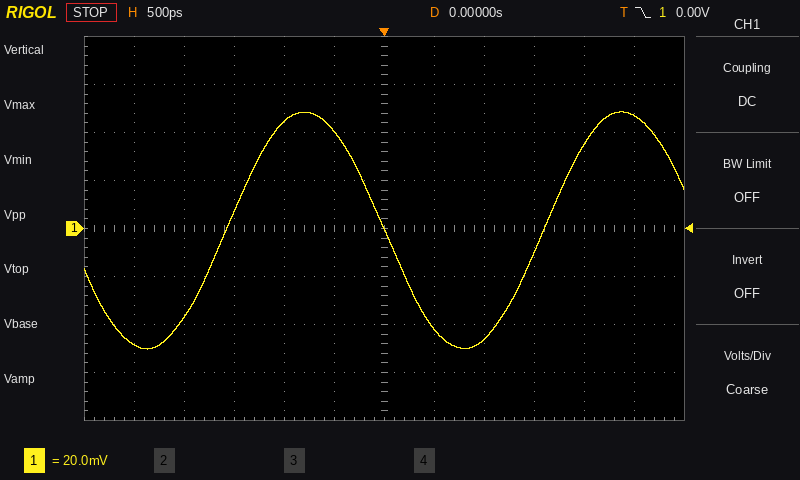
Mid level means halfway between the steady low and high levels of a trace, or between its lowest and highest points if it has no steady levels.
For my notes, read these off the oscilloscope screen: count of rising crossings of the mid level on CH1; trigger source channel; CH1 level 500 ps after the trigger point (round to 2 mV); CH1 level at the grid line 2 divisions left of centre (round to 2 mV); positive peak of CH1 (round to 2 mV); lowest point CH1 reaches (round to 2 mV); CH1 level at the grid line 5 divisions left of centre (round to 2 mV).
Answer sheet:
2
CH1
-42 mV
44 mV
48 mV
-50 mV
-48 mV
